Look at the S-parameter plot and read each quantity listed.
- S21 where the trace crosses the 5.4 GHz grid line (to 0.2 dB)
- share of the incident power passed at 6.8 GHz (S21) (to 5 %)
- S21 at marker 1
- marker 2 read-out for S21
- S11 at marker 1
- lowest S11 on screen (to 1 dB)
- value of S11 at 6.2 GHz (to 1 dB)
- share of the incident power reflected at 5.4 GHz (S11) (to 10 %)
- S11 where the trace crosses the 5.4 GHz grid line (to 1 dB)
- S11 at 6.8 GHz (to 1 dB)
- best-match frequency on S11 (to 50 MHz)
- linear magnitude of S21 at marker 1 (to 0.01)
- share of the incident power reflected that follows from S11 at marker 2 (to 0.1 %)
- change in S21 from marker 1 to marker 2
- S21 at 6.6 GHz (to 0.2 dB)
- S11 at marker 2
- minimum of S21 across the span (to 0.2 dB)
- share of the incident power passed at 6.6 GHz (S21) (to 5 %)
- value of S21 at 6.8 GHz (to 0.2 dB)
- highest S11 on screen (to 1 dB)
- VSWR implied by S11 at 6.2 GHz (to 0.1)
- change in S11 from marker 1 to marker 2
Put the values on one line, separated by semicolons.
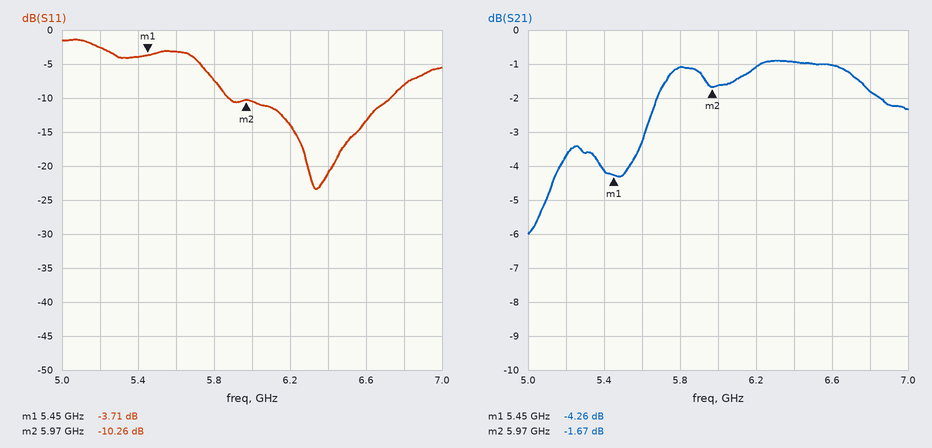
-4.2 dB; 65 %; -4.26 dB; -1.67 dB; -3.71 dB; -23 dB; -14 dB; 40 %; -4 dB; -8 dB; 6.35 GHz; 0.61; 9.4 %; 2.59 dB; -1.0 dB; -10.26 dB; -6.0 dB; 80 %; -1.8 dB; -1 dB; 1.5; -6.55 dB
